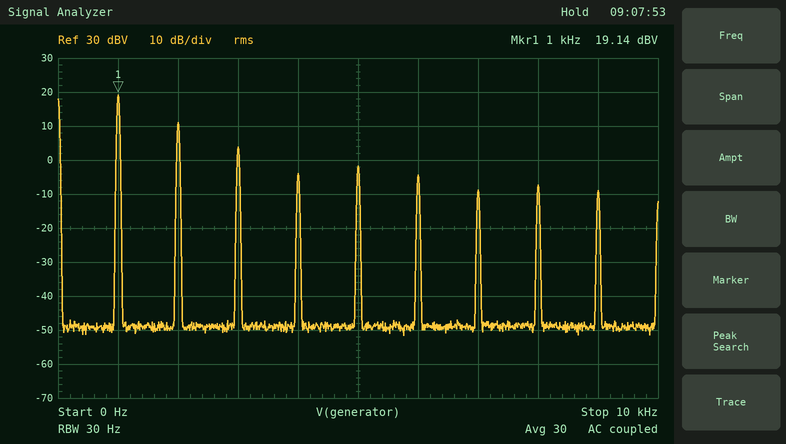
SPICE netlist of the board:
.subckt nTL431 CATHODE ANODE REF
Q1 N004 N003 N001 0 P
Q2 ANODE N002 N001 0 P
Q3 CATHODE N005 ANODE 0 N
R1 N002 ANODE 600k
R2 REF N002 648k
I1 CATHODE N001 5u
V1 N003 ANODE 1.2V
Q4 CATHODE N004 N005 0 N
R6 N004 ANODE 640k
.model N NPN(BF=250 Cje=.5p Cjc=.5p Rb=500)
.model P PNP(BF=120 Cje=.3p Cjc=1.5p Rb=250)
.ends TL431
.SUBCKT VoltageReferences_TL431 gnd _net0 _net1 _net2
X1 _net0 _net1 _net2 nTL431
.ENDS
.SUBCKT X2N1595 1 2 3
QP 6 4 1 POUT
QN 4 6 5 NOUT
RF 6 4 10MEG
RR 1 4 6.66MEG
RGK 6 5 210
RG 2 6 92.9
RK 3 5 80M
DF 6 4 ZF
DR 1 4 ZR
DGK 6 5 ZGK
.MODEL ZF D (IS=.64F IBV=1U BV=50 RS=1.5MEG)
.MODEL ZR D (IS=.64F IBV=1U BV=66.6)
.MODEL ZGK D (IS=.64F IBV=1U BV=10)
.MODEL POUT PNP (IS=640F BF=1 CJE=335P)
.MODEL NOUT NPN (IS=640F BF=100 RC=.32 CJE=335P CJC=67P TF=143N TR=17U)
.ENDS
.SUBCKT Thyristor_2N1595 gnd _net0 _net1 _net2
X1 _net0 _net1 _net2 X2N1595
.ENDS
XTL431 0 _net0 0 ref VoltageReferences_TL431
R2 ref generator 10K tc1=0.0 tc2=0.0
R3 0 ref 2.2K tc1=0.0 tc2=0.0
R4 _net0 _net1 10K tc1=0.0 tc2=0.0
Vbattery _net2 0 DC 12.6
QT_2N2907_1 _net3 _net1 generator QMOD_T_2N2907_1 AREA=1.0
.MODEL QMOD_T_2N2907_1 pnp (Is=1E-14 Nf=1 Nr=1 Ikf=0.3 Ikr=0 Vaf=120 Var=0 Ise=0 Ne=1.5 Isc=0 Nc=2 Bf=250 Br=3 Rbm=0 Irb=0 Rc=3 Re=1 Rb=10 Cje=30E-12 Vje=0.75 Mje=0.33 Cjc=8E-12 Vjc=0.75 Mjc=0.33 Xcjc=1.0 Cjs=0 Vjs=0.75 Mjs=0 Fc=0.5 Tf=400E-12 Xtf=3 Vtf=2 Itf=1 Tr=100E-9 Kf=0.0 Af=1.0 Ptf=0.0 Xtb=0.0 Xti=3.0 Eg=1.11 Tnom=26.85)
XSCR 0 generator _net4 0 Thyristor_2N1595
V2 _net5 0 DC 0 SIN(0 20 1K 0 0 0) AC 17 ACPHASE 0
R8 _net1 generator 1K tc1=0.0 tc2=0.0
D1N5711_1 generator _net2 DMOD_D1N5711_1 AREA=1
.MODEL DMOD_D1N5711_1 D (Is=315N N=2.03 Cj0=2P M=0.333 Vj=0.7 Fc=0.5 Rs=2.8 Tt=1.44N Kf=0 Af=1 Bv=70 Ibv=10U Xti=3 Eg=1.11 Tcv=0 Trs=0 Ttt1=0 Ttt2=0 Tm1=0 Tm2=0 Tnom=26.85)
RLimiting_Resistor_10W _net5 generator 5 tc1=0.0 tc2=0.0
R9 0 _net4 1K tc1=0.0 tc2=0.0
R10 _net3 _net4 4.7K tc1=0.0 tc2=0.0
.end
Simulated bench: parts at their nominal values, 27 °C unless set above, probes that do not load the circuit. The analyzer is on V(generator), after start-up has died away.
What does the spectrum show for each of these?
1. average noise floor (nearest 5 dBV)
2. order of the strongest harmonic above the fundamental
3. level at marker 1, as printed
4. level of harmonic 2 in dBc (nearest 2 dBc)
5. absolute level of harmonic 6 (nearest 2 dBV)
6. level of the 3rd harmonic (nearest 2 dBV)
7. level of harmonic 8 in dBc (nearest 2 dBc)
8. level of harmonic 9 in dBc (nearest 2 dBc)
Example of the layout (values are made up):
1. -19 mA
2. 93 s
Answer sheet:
1. -50 dBV
2. 2
3. 19.14 dBV
4. -8 dBc
5. -4 dBV
6. 4 dBV
7. -26 dBc
8. -28 dBc
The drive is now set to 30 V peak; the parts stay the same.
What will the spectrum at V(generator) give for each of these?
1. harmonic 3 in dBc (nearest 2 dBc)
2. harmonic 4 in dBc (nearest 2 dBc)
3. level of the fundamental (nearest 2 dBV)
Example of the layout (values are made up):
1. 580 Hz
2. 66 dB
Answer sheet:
1. -20 dBc
2. -20 dBc
3. 22 dBV
